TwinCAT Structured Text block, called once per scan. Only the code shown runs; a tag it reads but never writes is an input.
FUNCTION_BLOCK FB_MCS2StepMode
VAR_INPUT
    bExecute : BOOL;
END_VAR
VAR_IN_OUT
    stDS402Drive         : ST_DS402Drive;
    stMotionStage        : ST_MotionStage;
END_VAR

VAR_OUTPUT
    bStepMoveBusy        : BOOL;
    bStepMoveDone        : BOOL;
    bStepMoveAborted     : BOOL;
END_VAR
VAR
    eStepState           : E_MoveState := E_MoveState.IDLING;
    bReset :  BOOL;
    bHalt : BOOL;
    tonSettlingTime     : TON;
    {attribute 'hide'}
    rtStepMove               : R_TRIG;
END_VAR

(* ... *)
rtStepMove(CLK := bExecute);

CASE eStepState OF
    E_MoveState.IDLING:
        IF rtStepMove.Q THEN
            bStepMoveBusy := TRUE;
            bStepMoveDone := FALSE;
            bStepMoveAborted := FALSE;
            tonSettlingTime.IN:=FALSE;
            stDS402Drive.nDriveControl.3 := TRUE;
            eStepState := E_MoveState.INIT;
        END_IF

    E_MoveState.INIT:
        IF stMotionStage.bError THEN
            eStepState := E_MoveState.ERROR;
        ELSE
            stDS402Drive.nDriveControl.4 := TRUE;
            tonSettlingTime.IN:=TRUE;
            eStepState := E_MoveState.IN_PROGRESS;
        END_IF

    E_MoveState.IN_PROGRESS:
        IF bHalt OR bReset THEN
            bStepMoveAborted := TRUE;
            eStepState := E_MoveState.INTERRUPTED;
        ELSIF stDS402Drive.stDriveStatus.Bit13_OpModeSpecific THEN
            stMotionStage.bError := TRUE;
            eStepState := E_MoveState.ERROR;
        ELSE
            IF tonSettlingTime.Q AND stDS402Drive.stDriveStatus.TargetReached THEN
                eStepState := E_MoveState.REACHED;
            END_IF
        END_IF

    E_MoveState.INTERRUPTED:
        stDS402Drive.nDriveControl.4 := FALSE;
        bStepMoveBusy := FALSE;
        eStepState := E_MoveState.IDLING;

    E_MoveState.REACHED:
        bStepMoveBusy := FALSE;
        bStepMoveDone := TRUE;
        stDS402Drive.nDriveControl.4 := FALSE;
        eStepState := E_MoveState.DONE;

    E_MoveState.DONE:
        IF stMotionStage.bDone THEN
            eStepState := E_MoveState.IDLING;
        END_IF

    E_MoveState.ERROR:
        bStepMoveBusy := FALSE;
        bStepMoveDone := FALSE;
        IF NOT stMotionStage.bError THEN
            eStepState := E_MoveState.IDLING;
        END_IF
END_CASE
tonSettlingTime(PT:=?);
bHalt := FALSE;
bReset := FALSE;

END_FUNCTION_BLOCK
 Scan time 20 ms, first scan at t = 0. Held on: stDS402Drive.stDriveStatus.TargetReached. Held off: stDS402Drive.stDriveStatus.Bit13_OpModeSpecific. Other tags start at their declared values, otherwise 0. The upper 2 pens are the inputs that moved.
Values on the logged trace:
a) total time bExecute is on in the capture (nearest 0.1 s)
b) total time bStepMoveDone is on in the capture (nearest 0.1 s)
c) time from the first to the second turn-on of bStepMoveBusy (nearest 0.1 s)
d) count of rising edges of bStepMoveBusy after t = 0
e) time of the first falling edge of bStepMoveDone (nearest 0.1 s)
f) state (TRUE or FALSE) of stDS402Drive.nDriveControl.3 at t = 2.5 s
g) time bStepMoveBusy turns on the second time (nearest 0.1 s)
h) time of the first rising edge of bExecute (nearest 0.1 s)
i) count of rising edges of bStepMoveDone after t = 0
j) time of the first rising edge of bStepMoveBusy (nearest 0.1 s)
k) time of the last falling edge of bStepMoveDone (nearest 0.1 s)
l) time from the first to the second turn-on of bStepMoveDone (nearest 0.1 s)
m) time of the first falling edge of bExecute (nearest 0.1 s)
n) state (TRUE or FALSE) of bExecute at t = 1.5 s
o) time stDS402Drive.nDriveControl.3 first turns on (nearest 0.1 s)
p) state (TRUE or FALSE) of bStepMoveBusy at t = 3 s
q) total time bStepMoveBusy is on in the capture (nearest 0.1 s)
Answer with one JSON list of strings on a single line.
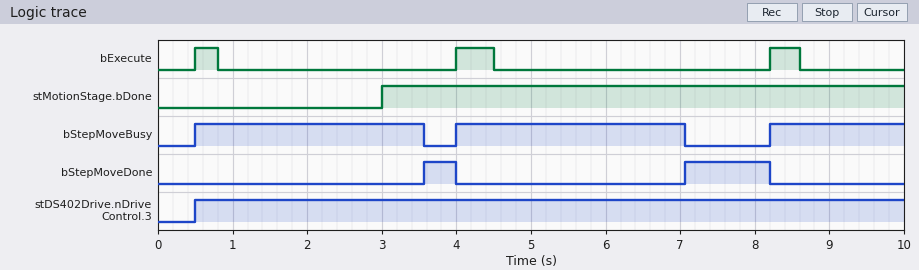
["1.2 s", "1.6 s", "3.5 s", "3", "4.0 s", "TRUE", "4.0 s", "0.5 s", "2", "0.5 s", "8.2 s", "3.5 s", "0.8 s", "FALSE", "0.5 s", "TRUE", "7.9 s"]
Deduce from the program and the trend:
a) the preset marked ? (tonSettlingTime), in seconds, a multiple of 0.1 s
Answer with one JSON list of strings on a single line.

["3.0 s"]
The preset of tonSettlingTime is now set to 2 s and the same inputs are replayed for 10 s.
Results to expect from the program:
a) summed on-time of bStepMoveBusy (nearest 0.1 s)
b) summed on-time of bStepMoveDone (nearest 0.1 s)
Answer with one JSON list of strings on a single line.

["5.9 s", "3.6 s"]
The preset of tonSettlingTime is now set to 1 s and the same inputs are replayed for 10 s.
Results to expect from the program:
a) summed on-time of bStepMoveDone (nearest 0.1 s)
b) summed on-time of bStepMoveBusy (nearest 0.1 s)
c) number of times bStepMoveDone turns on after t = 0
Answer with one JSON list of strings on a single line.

["6.3 s", "3.2 s", "3"]
